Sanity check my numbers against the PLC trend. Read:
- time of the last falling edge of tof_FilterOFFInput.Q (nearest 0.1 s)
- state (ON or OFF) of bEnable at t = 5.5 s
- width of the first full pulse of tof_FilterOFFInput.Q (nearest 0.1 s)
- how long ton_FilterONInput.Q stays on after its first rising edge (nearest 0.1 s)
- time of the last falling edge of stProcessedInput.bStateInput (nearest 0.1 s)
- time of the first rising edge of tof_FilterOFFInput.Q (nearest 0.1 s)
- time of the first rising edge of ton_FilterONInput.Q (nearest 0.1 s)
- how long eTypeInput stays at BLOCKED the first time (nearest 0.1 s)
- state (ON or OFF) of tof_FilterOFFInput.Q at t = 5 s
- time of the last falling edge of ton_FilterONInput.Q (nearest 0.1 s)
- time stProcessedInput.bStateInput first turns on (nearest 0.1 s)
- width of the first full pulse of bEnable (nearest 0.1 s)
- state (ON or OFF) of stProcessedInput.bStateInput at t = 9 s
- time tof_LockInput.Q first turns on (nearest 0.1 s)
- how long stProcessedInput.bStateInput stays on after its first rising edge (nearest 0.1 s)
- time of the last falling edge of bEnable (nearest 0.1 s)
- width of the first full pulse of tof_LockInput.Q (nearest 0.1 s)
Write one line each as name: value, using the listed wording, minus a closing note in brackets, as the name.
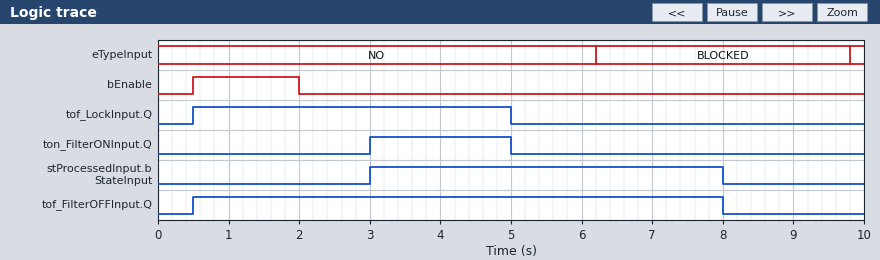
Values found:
time of the last falling edge of tof_FilterOFFInput.Q: 8.0 s
state (ON or OFF) of bEnable at t = 5.5 s: OFF
width of the first full pulse of tof_FilterOFFInput.Q: 7.5 s
how long ton_FilterONInput.Q stays on after its first rising edge: 2.0 s
time of the last falling edge of stProcessedInput.bStateInput: 8.0 s
time of the first rising edge of tof_FilterOFFInput.Q: 0.5 s
time of the first rising edge of ton_FilterONInput.Q: 3.0 s
how long eTypeInput stays at BLOCKED the first time: 3.6 s
state (ON or OFF) of tof_FilterOFFInput.Q at t = 5 s: ON
time of the last falling edge of ton_FilterONInput.Q: 5.0 s
time stProcessedInput.bStateInput first turns on: 3.0 s
width of the first full pulse of bEnable: 1.5 s
state (ON or OFF) of stProcessedInput.bStateInput at t = 9 s: OFF
time tof_LockInput.Q first turns on: 0.5 s
how long stProcessedInput.bStateInput stays on after its first rising edge: 5.0 s
time of the last falling edge of bEnable: 2.0 s
width of the first full pulse of tof_LockInput.Q: 4.5 s
